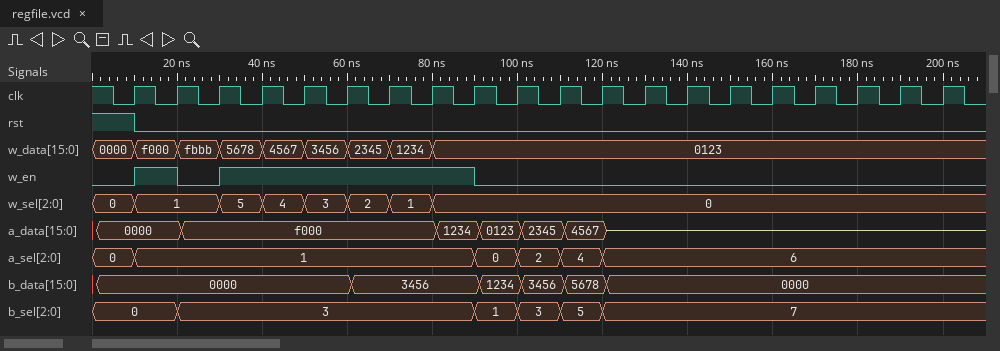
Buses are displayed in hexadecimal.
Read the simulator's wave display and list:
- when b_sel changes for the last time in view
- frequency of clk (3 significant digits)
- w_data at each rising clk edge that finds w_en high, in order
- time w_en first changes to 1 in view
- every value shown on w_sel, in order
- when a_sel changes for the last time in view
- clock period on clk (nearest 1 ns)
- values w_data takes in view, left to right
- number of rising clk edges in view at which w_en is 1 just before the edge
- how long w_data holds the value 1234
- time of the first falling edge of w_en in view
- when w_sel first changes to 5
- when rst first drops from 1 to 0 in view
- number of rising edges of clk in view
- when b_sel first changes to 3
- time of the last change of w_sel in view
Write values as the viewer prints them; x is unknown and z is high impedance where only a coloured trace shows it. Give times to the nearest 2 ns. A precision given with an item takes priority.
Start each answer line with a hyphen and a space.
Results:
- 120 ns
- 100 MHz
- f000, 5678, 4567, 3456, 2345, 1234, 0123
- 10 ns
- 0, 1, 5, 4, 3, 2, 1, 0
- 120 ns
- 10 ns
- 0000, f000, fbbb, 5678, 4567, 3456, 2345, 1234, 0123
- 7
- 10 ns
- 20 ns
- 30 ns
- 10 ns
- 20
- 20 ns
- 80 ns
